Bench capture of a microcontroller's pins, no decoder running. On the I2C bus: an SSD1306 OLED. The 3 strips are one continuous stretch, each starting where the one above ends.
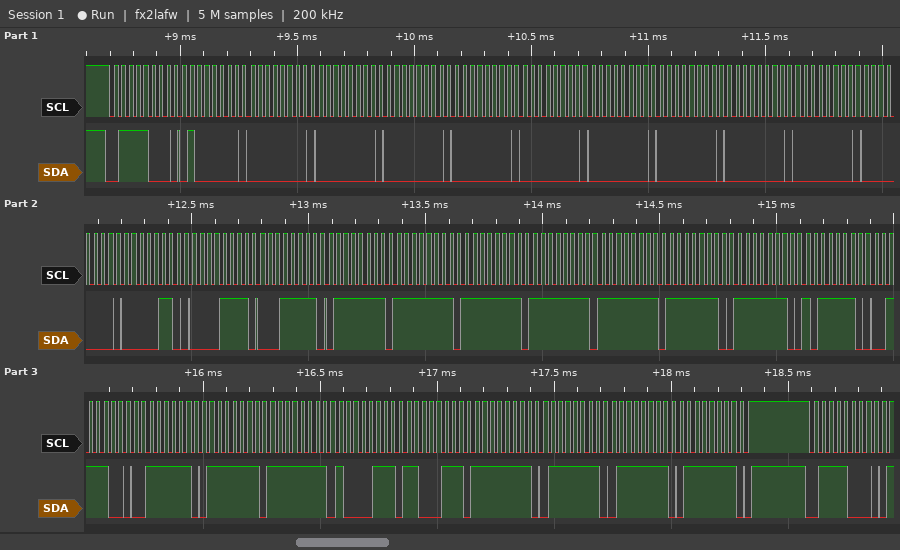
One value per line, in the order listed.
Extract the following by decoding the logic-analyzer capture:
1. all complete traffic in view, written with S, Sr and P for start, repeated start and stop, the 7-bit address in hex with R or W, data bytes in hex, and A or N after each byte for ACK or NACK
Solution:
S 3CW A 40 A 00 A 00 A 00 A 00 A 00 A 00 A 00 A 00 A 00 A 00 A 06 A 0F A 1F A 7F A FF A FF A FF A FF A FE A FE A BE A 3C A 3F A 7F A FF A 87 A C7 A FF A 7F A 7F A 7F A P S 3CW A
